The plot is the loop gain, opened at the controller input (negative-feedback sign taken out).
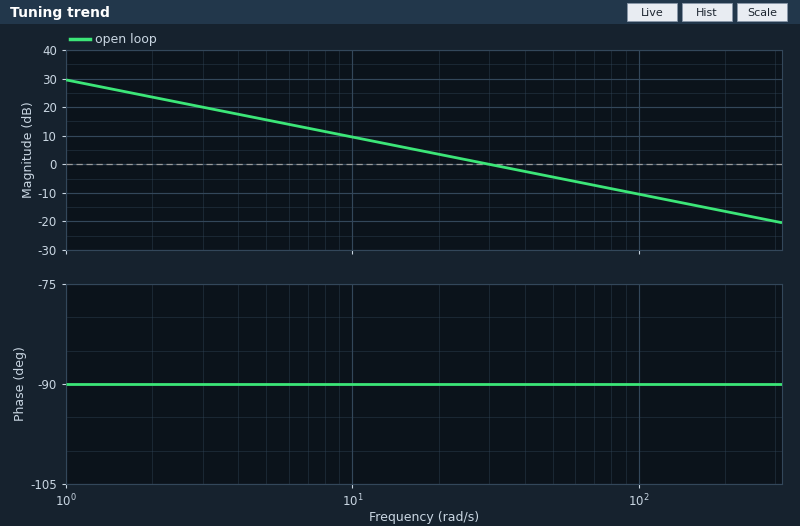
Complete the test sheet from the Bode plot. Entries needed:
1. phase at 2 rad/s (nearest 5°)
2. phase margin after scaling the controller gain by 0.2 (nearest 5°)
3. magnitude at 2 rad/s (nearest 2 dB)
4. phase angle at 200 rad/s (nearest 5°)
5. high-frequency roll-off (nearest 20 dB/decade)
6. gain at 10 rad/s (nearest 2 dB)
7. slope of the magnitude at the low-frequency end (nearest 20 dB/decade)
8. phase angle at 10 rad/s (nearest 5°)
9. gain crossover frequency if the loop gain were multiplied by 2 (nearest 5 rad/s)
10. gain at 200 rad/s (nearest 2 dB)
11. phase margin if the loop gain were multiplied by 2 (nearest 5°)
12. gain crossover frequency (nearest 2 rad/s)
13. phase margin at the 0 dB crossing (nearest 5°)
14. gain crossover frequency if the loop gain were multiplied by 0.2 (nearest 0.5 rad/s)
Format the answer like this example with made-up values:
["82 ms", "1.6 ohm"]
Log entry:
["-90°", "90°", "24 dB", "-90°", "-20 dB/decade", "10 dB", "-20 dB/decade", "-90°", "60 rad/s", "-16 dB", "90°", "30 rad/s", "90°", "6.0 rad/s"]
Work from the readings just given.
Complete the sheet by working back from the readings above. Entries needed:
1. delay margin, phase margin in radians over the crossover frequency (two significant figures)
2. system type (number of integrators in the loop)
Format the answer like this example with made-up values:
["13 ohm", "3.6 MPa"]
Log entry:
["0.052 s", "1"]
